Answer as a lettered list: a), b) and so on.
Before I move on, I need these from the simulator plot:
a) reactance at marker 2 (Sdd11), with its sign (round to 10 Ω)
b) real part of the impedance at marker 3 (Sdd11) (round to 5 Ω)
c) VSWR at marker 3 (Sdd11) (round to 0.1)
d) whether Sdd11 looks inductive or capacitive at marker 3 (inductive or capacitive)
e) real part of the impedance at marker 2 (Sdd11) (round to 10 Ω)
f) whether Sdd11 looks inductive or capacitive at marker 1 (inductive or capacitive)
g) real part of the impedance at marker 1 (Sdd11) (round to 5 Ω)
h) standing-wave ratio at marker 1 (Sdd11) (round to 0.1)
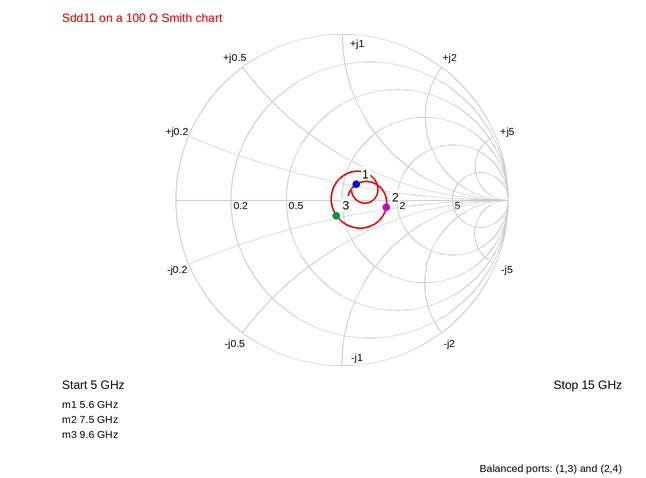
a) -20 Ω
b) 90 Ω
c) 1.2
d) capacitive
e) 170 Ω
f) inductive
g) 115 Ω
h) 1.3
